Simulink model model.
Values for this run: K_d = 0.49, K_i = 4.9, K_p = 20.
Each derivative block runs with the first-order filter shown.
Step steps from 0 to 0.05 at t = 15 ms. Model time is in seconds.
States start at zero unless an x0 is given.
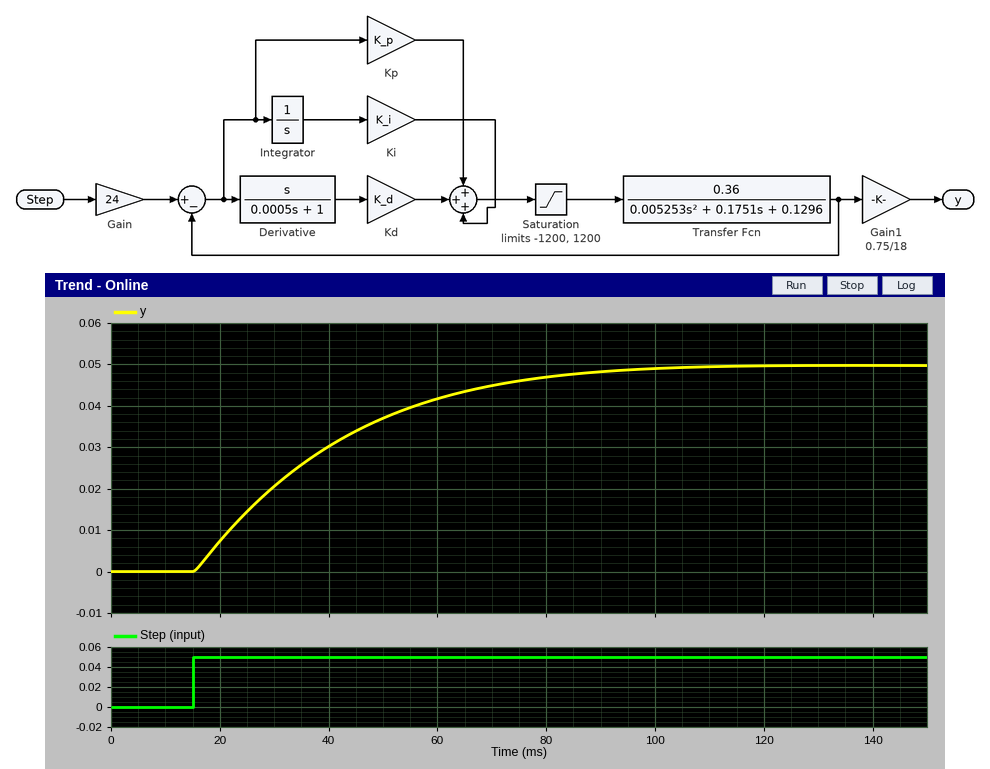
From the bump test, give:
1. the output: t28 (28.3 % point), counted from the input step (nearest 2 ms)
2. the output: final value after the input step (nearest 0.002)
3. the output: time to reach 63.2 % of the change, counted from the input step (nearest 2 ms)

10 ms
0.050
26 ms
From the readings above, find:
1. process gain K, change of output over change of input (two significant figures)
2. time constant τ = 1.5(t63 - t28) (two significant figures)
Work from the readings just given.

1.0
24 ms
